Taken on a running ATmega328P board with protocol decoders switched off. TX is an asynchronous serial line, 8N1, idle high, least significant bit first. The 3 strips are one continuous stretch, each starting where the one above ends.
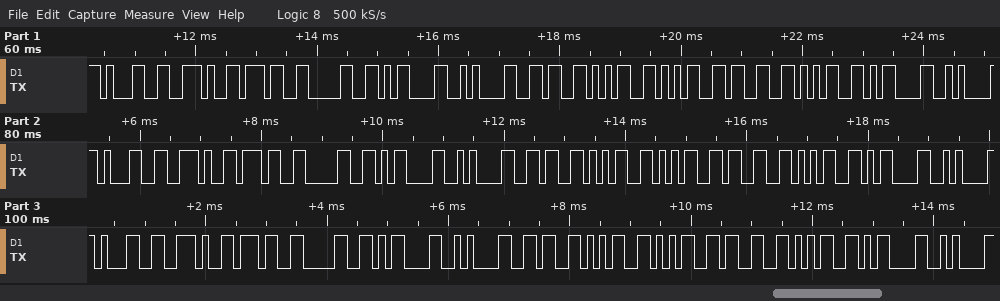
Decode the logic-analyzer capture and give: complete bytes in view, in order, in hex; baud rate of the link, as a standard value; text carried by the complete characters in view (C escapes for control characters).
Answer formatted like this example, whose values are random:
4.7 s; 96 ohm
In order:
31 2E 37 30 0D 0A 36 35 35 33 35 0D 0A 31 2E 37 30 0D 0A 36 35 35 33 35 0D 0A 31 2E 37 30 0D 0A 36 35 35 33 35 0D 0A; 9600 baud; "1.70\r\n65535\r\n1.70\r\n65535\r\n1.70\r\n65535\r\n"
